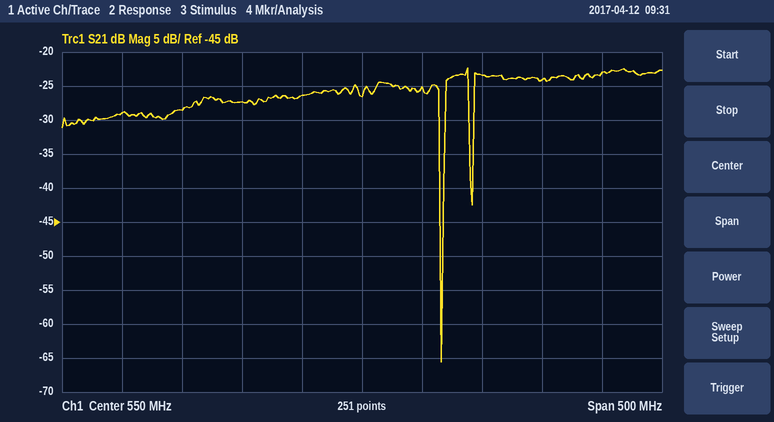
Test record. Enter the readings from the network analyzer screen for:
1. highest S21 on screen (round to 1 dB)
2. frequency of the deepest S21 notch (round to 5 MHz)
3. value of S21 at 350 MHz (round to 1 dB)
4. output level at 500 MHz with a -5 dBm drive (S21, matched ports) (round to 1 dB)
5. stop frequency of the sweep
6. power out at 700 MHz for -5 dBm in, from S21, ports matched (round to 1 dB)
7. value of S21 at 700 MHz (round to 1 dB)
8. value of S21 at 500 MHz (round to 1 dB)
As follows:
-22 dB
615 MHz
-29 dB
-31 dBm
800 MHz
-29 dBm
-24 dB
-26 dB
